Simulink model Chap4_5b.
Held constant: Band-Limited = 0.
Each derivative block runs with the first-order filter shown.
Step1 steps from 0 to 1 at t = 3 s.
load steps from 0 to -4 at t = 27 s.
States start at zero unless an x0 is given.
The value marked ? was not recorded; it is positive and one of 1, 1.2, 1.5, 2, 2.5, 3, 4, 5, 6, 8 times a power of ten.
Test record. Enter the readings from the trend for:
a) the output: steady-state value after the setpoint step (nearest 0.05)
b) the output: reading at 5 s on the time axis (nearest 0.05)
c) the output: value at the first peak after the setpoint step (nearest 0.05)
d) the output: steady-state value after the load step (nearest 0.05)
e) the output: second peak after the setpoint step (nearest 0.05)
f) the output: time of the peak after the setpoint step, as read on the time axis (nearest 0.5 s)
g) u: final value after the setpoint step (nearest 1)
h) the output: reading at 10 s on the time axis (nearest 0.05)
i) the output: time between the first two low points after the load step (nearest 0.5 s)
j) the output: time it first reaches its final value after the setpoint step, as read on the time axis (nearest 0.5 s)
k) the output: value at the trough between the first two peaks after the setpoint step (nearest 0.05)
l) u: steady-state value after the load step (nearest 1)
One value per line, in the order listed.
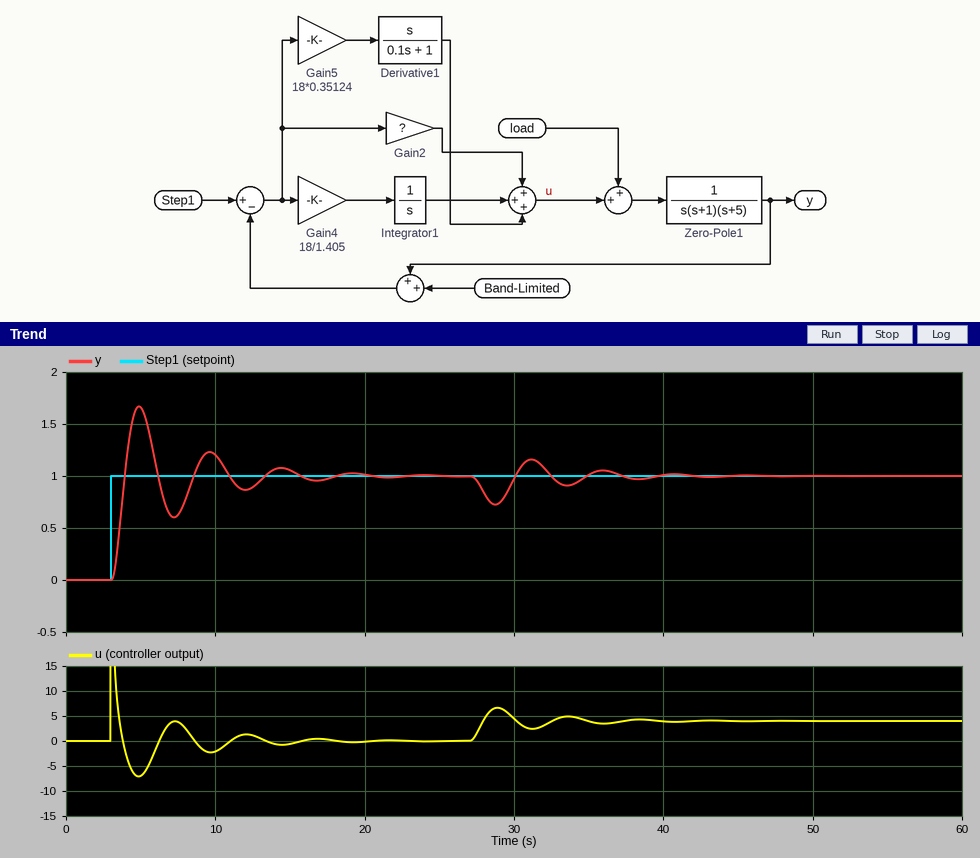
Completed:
1.00
1.65
1.65
1.00
1.25
5.0 s
0
1.20
5.0 s
4.0 s
0.60
4
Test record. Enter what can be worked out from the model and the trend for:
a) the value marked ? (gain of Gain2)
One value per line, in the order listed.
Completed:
12
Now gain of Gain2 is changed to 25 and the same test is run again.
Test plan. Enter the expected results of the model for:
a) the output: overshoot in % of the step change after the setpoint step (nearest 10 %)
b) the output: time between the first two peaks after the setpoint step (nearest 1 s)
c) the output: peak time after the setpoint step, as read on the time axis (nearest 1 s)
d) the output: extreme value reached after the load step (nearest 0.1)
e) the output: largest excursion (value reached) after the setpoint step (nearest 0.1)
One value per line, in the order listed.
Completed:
80 %
3 s
4 s
0.8
1.8
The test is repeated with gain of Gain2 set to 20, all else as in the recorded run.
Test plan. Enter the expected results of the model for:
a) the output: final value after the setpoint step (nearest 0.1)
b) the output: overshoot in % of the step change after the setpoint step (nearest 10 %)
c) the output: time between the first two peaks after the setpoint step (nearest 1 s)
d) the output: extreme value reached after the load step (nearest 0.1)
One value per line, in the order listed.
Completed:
1.0
70 %
3 s
0.8
